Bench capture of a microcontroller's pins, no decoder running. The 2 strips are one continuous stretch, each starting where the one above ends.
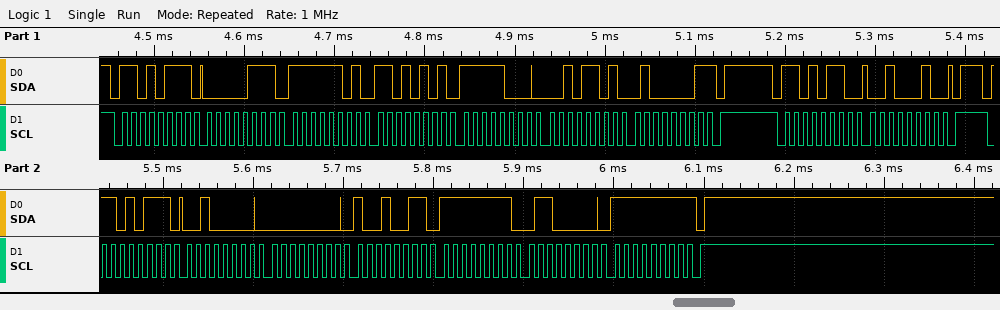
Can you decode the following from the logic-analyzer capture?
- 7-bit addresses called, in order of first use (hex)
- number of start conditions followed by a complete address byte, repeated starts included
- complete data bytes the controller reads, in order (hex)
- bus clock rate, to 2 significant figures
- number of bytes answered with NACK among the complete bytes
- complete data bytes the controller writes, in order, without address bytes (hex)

0x6B
3
07 FD D5 F8 2D 41 20 00 93 FF 60 FF
100 kHz
2
22
